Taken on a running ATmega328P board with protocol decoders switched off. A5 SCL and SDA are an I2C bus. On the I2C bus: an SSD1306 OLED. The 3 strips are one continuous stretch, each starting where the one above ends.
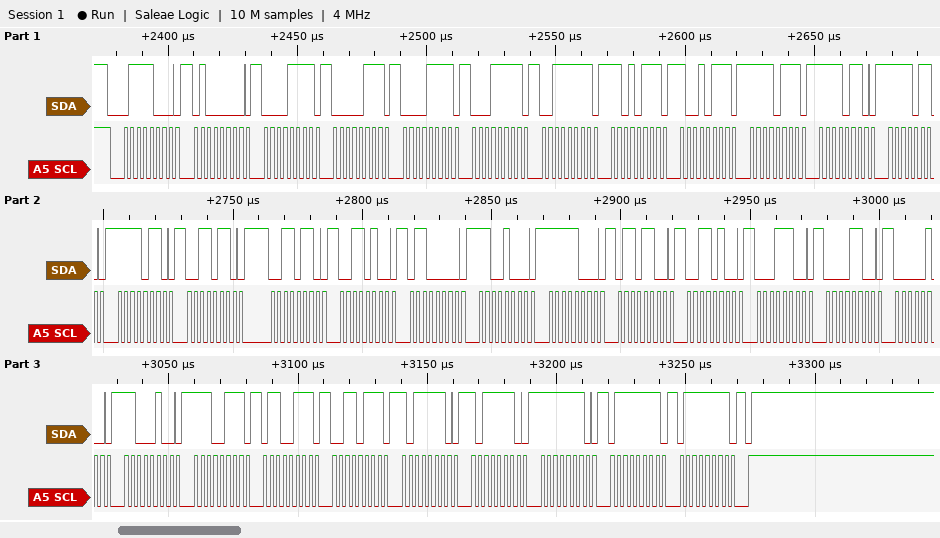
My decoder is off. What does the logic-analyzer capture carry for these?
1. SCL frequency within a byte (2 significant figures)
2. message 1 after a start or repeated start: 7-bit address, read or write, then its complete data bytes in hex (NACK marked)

400 kHz
0x3C write: 40 0F 07 0F 1F 3F D7 97 F7 F6 F6 F6 36 36 34 60 C8 F8 6C 34 1C 0C 04 C4 E7 67 37 BE BE FE 7F 7F
